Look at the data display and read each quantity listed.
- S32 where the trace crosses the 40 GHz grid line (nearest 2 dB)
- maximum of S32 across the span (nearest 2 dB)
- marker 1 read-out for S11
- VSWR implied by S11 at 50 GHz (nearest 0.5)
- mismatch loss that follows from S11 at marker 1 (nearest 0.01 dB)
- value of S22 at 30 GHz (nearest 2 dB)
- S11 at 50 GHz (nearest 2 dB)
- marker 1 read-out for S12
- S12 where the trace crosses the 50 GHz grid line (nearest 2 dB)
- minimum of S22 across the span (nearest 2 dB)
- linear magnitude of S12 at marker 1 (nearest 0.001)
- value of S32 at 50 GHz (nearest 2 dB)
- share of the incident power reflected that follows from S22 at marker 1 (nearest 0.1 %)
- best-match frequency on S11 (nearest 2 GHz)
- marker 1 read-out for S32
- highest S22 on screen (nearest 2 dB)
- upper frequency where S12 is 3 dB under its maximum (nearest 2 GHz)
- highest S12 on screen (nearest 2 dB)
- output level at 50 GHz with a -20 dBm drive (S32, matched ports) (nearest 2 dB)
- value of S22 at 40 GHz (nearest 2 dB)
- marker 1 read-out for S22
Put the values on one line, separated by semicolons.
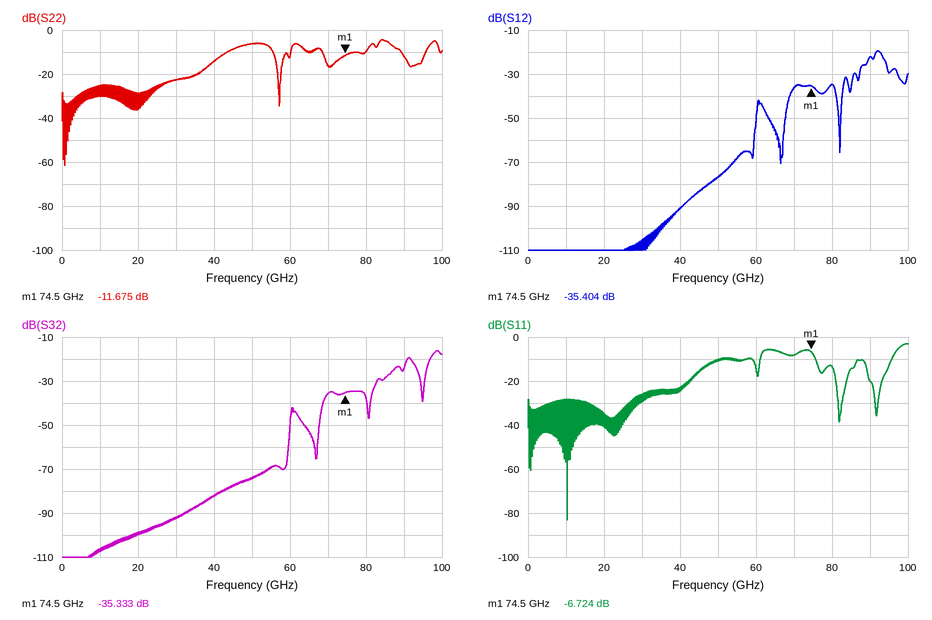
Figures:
-82 dB; -16 dB; -6.724 dB; 2.0; 1.04 dB; -22 dB; -10 dB; -35.404 dB; -76 dB; -62 dB; 0.017; -74 dB; 6.8 %; 10 GHz; -35.333 dB; -4 dB; 94 GHz; -20 dB; -94 dBm; -14 dB; -11.675 dB
